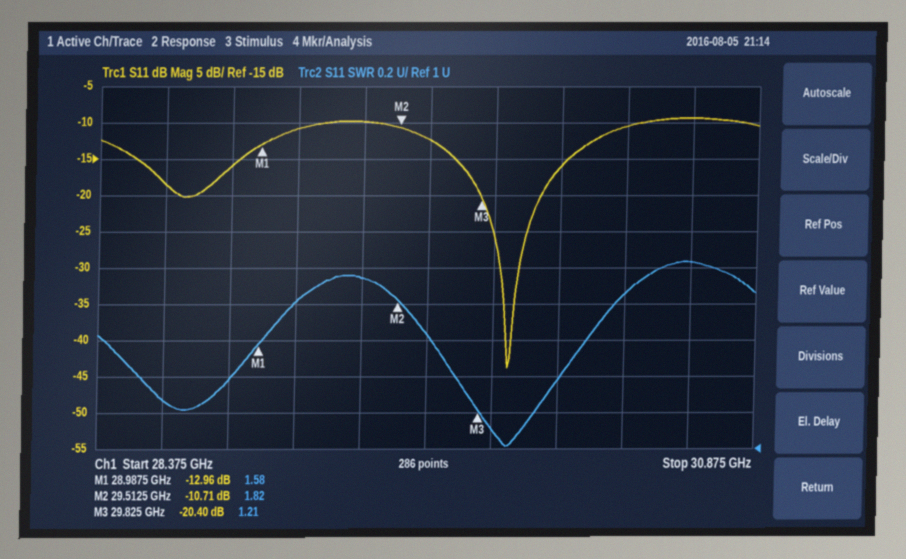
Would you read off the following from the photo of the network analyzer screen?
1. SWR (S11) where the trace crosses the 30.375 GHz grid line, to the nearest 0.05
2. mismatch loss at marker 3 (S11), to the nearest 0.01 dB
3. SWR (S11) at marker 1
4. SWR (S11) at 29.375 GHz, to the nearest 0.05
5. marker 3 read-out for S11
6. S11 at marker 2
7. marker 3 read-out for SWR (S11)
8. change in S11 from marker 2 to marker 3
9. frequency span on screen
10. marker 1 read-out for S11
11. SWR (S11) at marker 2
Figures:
1.85
0.04 dB
1.58
1.95
-20.40 dB
-10.71 dB
1.21
-9.69 dB
2.5 GHz
-12.96 dB
1.82
